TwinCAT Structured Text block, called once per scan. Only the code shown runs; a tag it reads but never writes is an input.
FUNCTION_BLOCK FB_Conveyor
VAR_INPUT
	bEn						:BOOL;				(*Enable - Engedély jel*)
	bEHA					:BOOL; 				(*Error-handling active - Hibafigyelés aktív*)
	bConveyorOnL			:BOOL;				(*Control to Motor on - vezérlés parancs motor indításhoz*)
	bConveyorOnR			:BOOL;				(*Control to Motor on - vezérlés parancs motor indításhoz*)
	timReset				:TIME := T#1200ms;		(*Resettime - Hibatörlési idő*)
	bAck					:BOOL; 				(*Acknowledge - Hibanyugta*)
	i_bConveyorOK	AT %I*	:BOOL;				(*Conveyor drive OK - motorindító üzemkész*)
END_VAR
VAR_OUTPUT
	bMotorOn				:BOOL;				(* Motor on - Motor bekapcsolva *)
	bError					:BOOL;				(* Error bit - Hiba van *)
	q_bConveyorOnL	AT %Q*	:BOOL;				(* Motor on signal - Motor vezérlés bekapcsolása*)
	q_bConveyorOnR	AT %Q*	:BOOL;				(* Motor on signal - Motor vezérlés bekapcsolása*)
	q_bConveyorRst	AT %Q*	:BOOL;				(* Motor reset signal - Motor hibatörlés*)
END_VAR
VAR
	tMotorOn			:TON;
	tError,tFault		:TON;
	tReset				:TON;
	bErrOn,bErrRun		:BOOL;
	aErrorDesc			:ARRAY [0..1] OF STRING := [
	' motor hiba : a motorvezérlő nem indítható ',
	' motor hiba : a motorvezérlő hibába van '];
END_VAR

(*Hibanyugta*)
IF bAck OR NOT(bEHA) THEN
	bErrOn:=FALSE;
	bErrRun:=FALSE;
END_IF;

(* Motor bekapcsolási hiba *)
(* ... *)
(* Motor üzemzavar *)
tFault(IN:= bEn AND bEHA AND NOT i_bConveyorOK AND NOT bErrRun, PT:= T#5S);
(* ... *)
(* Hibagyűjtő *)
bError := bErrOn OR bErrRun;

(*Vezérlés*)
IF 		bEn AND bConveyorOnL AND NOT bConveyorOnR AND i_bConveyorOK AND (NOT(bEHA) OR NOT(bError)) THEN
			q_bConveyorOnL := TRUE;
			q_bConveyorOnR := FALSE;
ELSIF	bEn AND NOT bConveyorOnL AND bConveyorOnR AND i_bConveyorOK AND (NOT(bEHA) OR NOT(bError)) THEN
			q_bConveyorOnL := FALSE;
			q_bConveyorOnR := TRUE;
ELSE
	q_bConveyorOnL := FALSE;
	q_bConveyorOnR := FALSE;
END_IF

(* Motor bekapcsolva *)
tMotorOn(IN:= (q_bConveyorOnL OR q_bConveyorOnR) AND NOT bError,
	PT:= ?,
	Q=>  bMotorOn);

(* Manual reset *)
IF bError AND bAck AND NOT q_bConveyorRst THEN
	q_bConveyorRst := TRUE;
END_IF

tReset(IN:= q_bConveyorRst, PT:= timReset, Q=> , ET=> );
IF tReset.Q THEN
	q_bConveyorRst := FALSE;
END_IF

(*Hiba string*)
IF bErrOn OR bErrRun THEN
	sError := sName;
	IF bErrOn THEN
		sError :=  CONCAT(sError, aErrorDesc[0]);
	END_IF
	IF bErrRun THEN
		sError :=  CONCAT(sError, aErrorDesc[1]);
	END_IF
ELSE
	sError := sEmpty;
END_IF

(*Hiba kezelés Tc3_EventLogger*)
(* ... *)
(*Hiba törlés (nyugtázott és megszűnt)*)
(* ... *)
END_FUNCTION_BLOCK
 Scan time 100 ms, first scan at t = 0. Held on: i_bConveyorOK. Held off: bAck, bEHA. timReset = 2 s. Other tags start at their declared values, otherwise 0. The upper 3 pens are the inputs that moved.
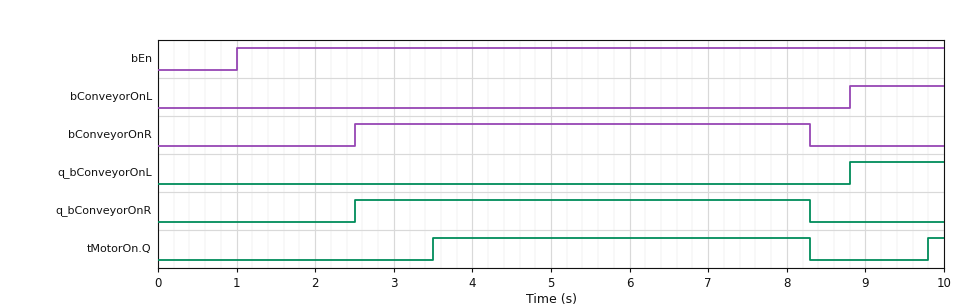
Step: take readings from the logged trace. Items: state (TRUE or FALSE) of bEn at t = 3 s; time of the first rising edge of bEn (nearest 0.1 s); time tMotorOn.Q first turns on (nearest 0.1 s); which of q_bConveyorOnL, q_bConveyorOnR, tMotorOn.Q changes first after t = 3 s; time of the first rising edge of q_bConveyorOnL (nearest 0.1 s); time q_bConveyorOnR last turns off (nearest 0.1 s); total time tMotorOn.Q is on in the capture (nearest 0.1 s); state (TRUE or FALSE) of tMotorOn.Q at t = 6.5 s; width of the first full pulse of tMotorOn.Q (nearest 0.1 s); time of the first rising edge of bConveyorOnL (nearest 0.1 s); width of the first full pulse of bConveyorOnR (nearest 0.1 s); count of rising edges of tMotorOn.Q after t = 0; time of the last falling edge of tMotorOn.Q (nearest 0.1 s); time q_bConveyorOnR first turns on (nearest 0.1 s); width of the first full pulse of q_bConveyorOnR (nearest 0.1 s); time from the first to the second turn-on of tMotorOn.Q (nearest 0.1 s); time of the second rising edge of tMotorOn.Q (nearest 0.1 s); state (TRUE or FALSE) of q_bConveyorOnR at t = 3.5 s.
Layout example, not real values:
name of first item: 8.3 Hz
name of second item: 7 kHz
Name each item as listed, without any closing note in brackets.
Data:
state (TRUE or FALSE) of bEn at t = 3 s: TRUE
time of the first rising edge of bEn: 1.0 s
time tMotorOn.Q first turns on: 3.5 s
which of q_bConveyorOnL, q_bConveyorOnR, tMotorOn.Q changes first after t = 3 s: tMotorOn.Q
time of the first rising edge of q_bConveyorOnL: 8.8 s
time q_bConveyorOnR last turns off: 8.3 s
total time tMotorOn.Q is on in the capture: 5.0 s
state (TRUE or FALSE) of tMotorOn.Q at t = 6.5 s: TRUE
width of the first full pulse of tMotorOn.Q: 4.8 s
time of the first rising edge of bConveyorOnL: 8.8 s
width of the first full pulse of bConveyorOnR: 5.8 s
count of rising edges of tMotorOn.Q after t = 0: 2
time of the last falling edge of tMotorOn.Q: 8.3 s
time q_bConveyorOnR first turns on: 2.5 s
width of the first full pulse of q_bConveyorOnR: 5.8 s
time from the first to the second turn-on of tMotorOn.Q: 6.3 s
time of the second rising edge of tMotorOn.Q: 9.8 s
state (TRUE or FALSE) of q_bConveyorOnR at t = 3.5 s: TRUE
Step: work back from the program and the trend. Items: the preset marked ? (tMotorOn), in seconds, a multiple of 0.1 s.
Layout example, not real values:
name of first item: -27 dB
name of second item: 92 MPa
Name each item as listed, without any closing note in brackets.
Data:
the preset marked ? (tMotorOn), in seconds, a multiple of 0.1 s: 1.0 s
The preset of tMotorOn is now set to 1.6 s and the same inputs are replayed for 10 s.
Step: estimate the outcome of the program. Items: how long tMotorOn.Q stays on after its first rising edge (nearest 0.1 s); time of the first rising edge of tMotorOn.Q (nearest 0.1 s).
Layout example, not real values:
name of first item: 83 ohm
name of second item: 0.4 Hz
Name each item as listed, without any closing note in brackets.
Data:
how long tMotorOn.Q stays on after its first rising edge: 4.2 s
time of the first rising edge of tMotorOn.Q: 4.1 s
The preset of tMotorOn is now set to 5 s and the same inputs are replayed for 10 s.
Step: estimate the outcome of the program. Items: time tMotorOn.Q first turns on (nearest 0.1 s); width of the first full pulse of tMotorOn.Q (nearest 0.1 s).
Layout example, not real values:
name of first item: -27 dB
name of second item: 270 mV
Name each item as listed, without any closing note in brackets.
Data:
time tMotorOn.Q first turns on: 7.5 s
width of the first full pulse of tMotorOn.Q: 0.8 s
